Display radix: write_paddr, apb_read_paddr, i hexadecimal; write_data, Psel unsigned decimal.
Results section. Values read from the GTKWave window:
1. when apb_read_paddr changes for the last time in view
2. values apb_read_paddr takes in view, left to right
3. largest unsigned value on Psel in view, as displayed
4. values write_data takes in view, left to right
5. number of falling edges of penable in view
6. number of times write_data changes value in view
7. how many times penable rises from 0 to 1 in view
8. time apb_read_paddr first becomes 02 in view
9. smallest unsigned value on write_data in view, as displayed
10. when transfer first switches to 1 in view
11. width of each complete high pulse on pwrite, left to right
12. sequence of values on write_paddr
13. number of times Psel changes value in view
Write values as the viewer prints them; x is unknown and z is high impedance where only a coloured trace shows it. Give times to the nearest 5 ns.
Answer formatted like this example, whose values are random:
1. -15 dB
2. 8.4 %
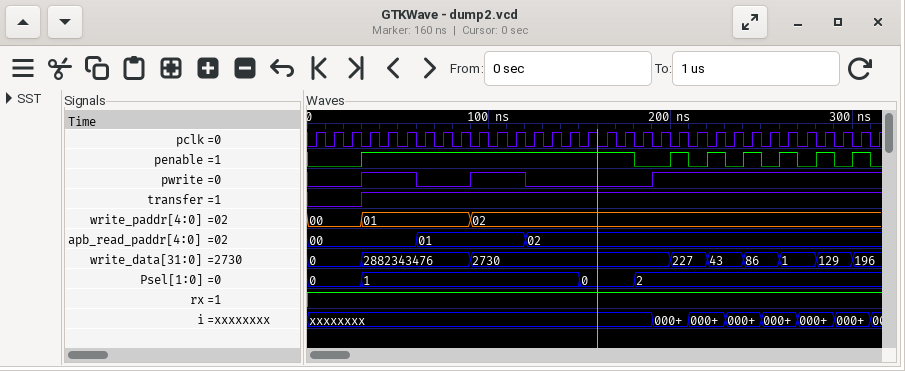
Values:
1. 120 ns
2. 00, 01, 02
3. 2
4. 0, 2882343476, 2730, 227, 43, 86, 1, 129, 196
5. 7
6. 8
7. 7
8. 120 ns
9. 0
10. 30 ns
11. 30 ns, 30 ns
12. 00, 01, 02
13. 3
